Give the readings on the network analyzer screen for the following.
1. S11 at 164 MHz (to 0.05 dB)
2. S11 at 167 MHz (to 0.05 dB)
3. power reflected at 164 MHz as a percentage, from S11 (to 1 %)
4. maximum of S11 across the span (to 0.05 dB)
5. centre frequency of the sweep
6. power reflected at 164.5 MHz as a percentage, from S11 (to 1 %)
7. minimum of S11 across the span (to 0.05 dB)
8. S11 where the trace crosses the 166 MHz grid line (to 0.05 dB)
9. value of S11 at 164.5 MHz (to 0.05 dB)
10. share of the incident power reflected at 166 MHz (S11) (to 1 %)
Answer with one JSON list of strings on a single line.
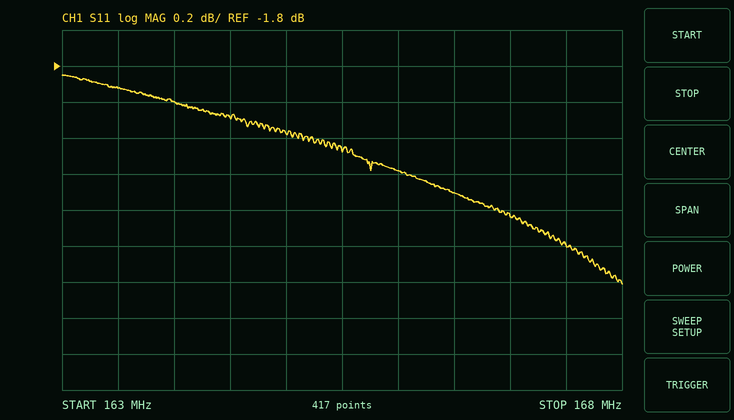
["-2.00 dB", "-2.65 dB", "63 %", "-1.85 dB", "165.5 MHz", "62 %", "-3.00 dB", "-2.40 dB", "-2.10 dB", "58 %"]
